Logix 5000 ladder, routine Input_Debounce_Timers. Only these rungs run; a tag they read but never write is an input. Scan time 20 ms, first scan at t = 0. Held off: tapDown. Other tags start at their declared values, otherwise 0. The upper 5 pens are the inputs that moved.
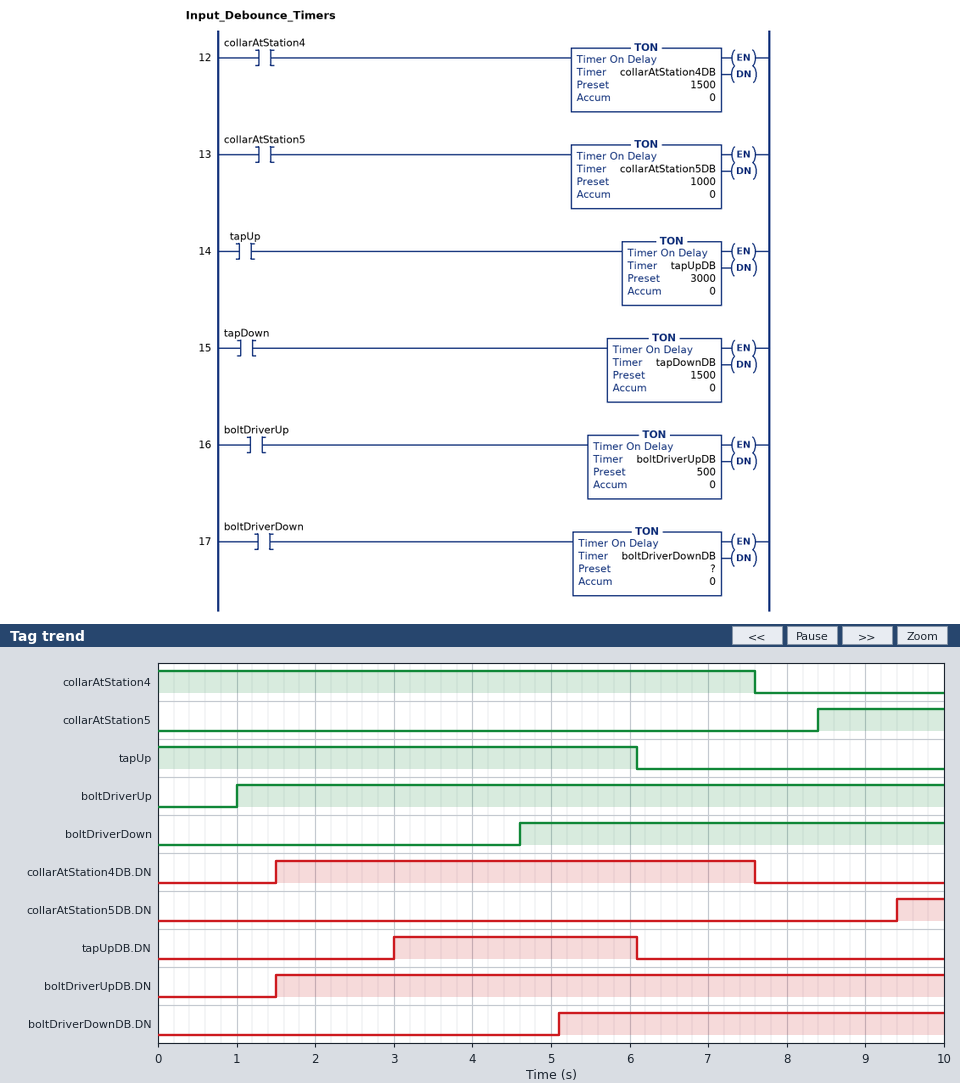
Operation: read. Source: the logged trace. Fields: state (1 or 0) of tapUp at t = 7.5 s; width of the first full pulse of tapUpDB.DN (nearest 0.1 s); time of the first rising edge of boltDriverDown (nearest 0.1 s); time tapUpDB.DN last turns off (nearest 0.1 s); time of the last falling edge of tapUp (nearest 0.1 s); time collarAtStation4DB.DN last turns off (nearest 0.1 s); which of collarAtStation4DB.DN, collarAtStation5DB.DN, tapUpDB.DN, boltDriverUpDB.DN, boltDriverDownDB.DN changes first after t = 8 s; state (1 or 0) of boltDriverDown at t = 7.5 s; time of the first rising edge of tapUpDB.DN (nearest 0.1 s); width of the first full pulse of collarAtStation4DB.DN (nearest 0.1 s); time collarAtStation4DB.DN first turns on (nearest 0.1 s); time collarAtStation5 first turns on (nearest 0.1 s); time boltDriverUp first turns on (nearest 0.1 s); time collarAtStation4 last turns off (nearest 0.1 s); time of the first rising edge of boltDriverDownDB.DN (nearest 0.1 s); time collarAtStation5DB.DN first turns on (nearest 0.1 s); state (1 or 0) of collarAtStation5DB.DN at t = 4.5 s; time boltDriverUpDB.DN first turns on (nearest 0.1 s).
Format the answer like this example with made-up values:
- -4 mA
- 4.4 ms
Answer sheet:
- 0
- 3.1 s
- 4.6 s
- 6.1 s
- 6.1 s
- 7.6 s
- collarAtStation5DB.DN
- 1
- 3.0 s
- 6.1 s
- 1.5 s
- 8.4 s
- 1.0 s
- 7.6 s
- 5.1 s
- 9.4 s
- 0
- 1.5 s
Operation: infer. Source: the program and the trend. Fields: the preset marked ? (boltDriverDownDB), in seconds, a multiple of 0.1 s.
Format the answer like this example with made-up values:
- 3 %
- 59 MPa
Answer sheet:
- 0.5 s
